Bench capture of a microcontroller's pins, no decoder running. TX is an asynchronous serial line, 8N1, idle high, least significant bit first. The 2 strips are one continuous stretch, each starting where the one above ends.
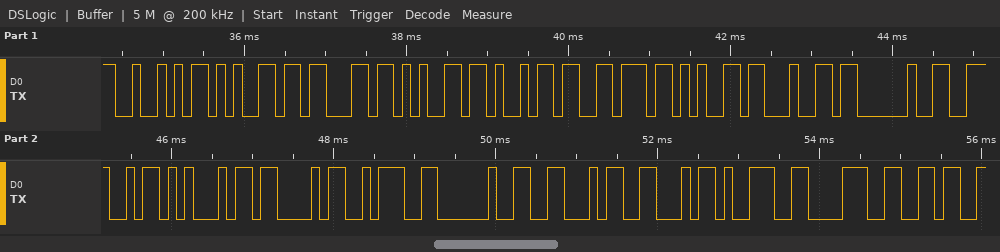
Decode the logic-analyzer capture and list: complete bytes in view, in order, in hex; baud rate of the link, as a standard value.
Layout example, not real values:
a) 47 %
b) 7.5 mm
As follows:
a) 0x52 0x65 0x63 0x65 0x69 0x76 0x65 0x64 0x20 0x4E 0x45 0x43 0x3A 0x20 0x46 0x46 0x39 0x38 0x36
b) 9600 baud
